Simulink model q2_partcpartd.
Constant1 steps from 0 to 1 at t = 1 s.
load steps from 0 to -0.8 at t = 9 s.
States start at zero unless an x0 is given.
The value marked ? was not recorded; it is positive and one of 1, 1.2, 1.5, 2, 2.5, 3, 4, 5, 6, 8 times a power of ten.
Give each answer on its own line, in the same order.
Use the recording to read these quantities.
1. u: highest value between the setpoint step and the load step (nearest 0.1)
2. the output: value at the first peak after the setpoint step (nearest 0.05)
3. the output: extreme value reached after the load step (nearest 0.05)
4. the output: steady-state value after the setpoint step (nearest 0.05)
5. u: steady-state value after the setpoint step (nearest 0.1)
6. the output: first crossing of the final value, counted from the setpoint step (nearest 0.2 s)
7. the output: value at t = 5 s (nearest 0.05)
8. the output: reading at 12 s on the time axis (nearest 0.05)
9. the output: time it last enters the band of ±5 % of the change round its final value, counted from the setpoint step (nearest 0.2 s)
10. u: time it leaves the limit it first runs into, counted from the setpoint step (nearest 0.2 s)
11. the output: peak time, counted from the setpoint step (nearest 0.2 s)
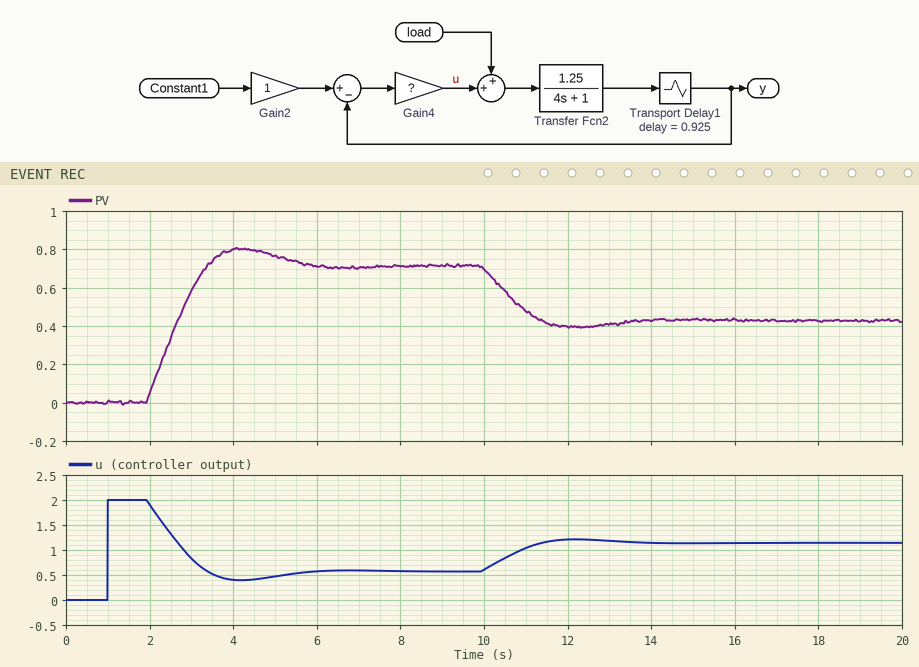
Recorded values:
2.0
0.80
0.40
0.70
0.6
2.4 s
0.75
0.40
4.2 s
1.0 s
3.2 s
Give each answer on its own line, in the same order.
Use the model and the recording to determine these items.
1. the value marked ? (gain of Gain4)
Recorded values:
2
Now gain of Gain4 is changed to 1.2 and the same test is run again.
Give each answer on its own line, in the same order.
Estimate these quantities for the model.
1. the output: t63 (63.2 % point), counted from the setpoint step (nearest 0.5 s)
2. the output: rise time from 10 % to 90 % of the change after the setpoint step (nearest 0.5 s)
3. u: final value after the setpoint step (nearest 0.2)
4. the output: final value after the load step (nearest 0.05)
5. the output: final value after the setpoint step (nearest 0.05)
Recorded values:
2.0 s
2.0 s
0.4
0.20
0.60
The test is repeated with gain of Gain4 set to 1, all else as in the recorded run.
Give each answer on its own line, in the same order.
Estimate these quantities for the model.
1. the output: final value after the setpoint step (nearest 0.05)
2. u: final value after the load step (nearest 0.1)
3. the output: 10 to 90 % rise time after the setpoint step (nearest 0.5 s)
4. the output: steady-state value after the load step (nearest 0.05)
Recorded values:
0.55
0.9
2.5 s
0.10
